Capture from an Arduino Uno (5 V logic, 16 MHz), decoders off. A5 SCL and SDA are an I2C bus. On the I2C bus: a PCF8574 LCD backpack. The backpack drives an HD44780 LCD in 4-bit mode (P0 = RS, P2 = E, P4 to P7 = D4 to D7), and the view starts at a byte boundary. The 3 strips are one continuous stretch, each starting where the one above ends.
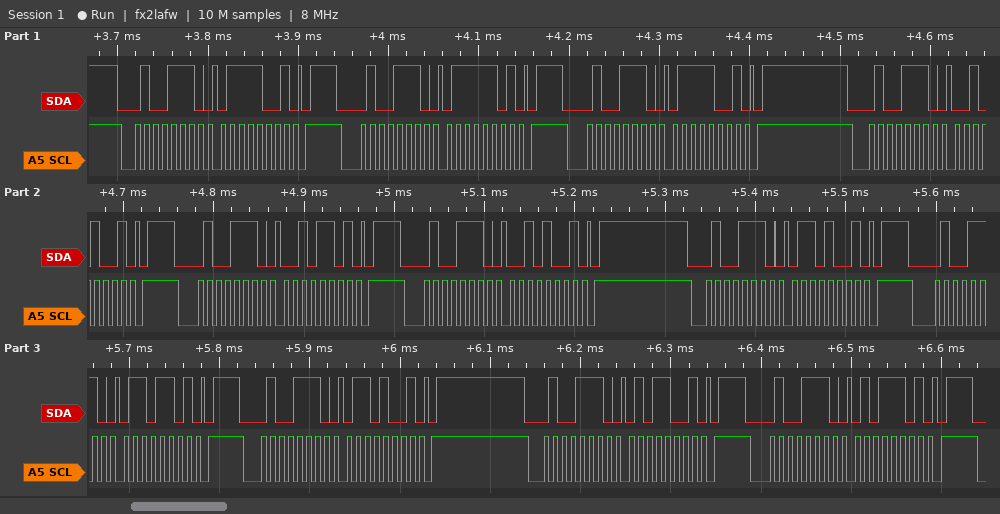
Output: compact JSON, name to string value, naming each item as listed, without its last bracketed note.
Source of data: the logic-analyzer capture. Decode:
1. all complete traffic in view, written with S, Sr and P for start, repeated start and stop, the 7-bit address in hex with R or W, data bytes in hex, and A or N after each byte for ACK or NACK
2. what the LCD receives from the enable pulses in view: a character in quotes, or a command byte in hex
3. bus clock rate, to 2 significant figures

{"all complete traffic in view, written with S, Sr and P for start, repeated start and stop, the 7-bit address in hex with R or W, data bytes in hex, and A or N after each byte for ACK or NACK": "S 27W A 79 A P S 27W A 7D A P S 27W A 79 A P S 27W A 29 A P S 27W A 2D A P S 27W A 29 A P S 27W A 69 A P S 27W A 6D A P S 27W A 69 A P S 27W A 59 A P S 27W A 5D A P", "what the LCD receives from the enable pulses in view: a character in quotes, or a command byte in hex": "'r'", "bus clock rate, to 2 significant figures": "100 kHz"}
